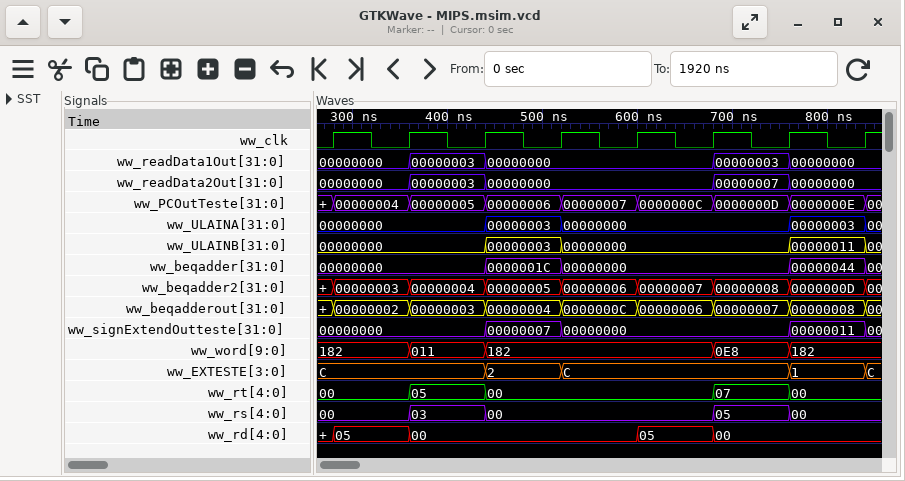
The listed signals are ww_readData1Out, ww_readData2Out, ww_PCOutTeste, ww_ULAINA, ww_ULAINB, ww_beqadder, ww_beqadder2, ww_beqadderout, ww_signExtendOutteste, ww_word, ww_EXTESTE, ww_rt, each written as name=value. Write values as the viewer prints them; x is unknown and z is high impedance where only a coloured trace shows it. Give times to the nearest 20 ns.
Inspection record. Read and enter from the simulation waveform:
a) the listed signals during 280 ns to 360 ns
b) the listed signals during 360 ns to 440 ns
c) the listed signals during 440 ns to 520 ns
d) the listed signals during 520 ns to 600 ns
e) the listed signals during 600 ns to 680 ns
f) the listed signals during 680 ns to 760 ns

ww_readData1Out=00000000, ww_readData2Out=00000000, ww_PCOutTeste=00000004, ww_ULAINA=00000000, ww_ULAINB=00000000, ww_beqadder=00000000, ww_beqadder2=00000003, ww_beqadderout=00000002, ww_signExtendOutteste=00000000, ww_word=182, ww_EXTESTE=C, ww_rt=00
ww_readData1Out=00000003, ww_readData2Out=00000003, ww_PCOutTeste=00000005, ww_ULAINA=00000000, ww_ULAINB=00000000, ww_beqadder=00000000, ww_beqadder2=00000004, ww_beqadderout=00000003, ww_signExtendOutteste=00000000, ww_word=011, ww_EXTESTE=C, ww_rt=05
ww_readData1Out=00000000, ww_readData2Out=00000000, ww_PCOutTeste=00000006, ww_ULAINA=00000003, ww_ULAINB=00000003, ww_beqadder=0000001C, ww_beqadder2=00000005, ww_beqadderout=00000004, ww_signExtendOutteste=00000007, ww_word=182, ww_EXTESTE=2, ww_rt=00
ww_readData1Out=00000000, ww_readData2Out=00000000, ww_PCOutTeste=00000007, ww_ULAINA=00000000, ww_ULAINB=00000000, ww_beqadder=00000000, ww_beqadder2=00000006, ww_beqadderout=0000000C, ww_signExtendOutteste=00000000, ww_word=182, ww_EXTESTE=C, ww_rt=00
ww_readData1Out=00000000, ww_readData2Out=00000000, ww_PCOutTeste=0000000C, ww_ULAINA=00000000, ww_ULAINB=00000000, ww_beqadder=00000000, ww_beqadder2=00000007, ww_beqadderout=00000006, ww_signExtendOutteste=00000000, ww_word=182, ww_EXTESTE=C, ww_rt=00
ww_readData1Out=00000003, ww_readData2Out=00000007, ww_PCOutTeste=0000000D, ww_ULAINA=00000000, ww_ULAINB=00000000, ww_beqadder=00000000, ww_beqadder2=00000008, ww_beqadderout=00000007, ww_signExtendOutteste=00000000, ww_word=0E8, ww_EXTESTE=C, ww_rt=07
